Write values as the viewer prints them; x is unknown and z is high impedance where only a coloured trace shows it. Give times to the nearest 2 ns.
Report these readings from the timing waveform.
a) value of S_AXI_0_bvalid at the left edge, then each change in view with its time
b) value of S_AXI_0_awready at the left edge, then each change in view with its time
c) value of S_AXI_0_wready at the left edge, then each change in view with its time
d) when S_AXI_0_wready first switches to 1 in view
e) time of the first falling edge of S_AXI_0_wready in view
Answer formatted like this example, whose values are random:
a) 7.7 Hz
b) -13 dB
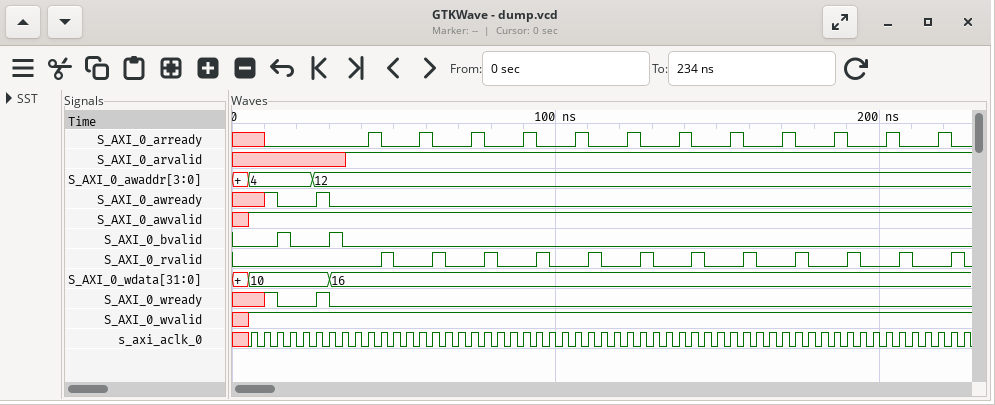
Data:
a) 0, 1 at 14 ns, 0 at 18 ns, 1 at 30 ns, 0 at 34 ns
b) x, 1 at 10 ns, 0 at 14 ns, 1 at 26 ns, 0 at 30 ns
c) x, 1 at 10 ns, 0 at 14 ns, 1 at 26 ns, 0 at 30 ns
d) 10 ns
e) 14 ns
